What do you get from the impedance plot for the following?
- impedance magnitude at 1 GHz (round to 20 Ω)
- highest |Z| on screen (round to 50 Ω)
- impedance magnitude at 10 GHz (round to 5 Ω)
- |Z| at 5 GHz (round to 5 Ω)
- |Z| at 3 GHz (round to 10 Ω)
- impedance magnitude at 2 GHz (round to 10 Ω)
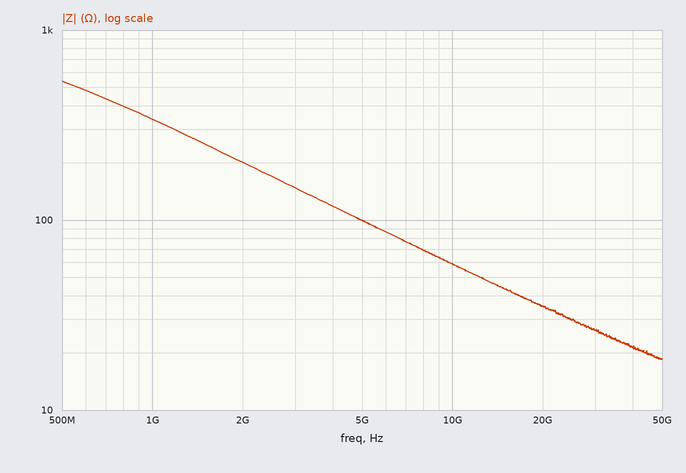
340 Ω
550 Ω
60 Ω
100 Ω
150 Ω
200 Ω
